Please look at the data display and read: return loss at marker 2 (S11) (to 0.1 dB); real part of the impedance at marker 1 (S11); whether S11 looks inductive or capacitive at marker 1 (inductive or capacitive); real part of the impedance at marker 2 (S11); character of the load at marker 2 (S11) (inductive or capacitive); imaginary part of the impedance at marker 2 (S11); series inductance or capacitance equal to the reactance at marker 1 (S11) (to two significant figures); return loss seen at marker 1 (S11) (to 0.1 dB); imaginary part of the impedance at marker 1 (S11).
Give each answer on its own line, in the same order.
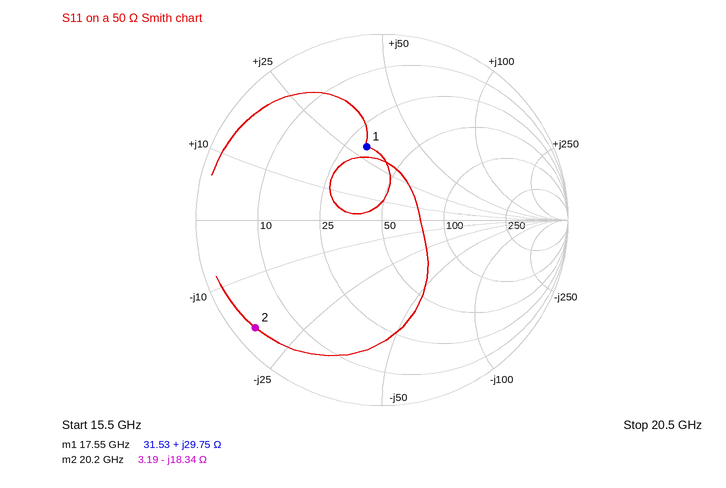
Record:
1.0 dB
31.53 Ω
inductive
3.19 Ω
capacitive
-18.34 Ω
270 pH
7.9 dB
+29.75 Ω
